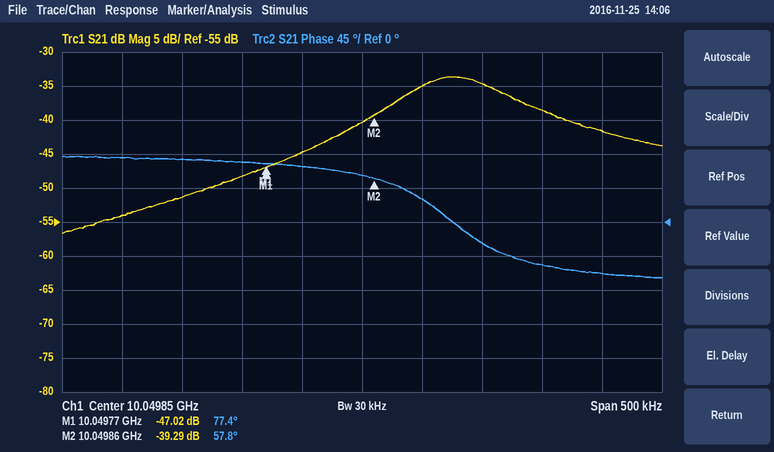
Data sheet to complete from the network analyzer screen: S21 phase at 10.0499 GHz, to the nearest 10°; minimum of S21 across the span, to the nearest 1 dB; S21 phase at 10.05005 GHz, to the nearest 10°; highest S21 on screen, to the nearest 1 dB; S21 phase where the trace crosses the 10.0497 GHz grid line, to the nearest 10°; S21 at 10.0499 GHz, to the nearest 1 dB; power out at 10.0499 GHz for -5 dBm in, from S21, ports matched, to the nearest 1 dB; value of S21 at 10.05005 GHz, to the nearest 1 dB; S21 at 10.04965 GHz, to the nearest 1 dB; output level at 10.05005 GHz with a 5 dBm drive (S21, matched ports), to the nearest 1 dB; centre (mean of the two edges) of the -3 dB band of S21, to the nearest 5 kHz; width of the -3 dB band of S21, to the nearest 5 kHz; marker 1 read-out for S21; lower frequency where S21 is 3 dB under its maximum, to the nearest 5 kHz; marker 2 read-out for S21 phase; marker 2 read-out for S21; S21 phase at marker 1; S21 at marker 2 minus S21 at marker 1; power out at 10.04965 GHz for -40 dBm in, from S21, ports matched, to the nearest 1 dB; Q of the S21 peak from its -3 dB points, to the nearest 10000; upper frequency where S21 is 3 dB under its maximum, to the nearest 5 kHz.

30°
-57 dB
-70°
-34 dB
80°
-35 dB
-40 dBm
-42 dB
-54 dB
-37 dBm
10.049930 GHz
90 kHz
-47.02 dB
10.049885 GHz
57.8°
-39.29 dB
77.4°
7.73 dB
-94 dBm
110000
10.049975 GHz
